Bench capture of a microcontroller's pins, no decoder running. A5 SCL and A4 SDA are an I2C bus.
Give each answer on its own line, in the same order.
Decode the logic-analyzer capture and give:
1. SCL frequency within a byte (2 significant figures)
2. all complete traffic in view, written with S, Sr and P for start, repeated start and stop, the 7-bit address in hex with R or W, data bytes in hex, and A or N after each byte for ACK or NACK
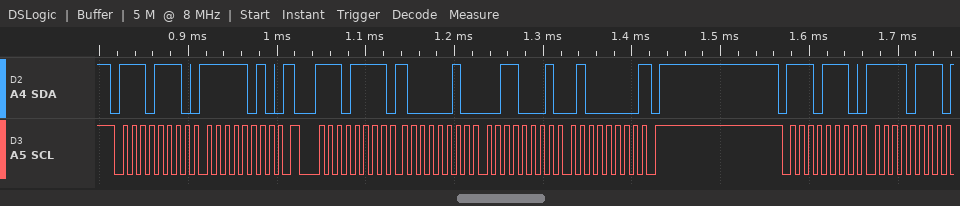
100 kHz
S 77W A FA A Sr 77R A 82 A 31 A 40 N P S 77W A F7 A
